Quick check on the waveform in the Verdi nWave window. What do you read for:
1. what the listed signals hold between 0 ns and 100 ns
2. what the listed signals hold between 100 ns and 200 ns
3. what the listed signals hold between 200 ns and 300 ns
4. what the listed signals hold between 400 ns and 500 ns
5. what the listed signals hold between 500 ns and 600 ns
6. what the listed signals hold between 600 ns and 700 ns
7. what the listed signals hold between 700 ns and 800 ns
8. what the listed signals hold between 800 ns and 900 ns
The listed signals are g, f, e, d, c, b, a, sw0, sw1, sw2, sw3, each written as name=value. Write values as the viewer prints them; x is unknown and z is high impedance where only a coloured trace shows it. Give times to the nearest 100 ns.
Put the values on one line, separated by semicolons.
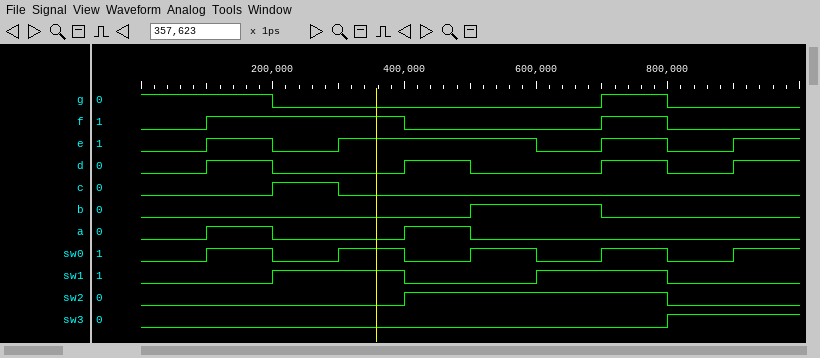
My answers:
g=1, f=0, e=0, d=0, c=0, b=0, a=0, sw0=0, sw1=0, sw2=0, sw3=0; g=1, f=1, e=1, d=1, c=0, b=0, a=1, sw0=1, sw1=0, sw2=0, sw3=0; g=0, f=1, e=0, d=0, c=1, b=0, a=0, sw0=0, sw1=1, sw2=0, sw3=0; g=0, f=0, e=1, d=1, c=0, b=0, a=1, sw0=0, sw1=0, sw2=1, sw3=0; g=0, f=0, e=1, d=0, c=0, b=1, a=0, sw0=1, sw1=0, sw2=1, sw3=0; g=0, f=0, e=0, d=0, c=0, b=1, a=0, sw0=0, sw1=1, sw2=1, sw3=0; g=1, f=1, e=1, d=1, c=0, b=0, a=0, sw0=1, sw1=1, sw2=1, sw3=0; g=0, f=0, e=0, d=0, c=0, b=0, a=0, sw0=0, sw1=0, sw2=0, sw3=1
